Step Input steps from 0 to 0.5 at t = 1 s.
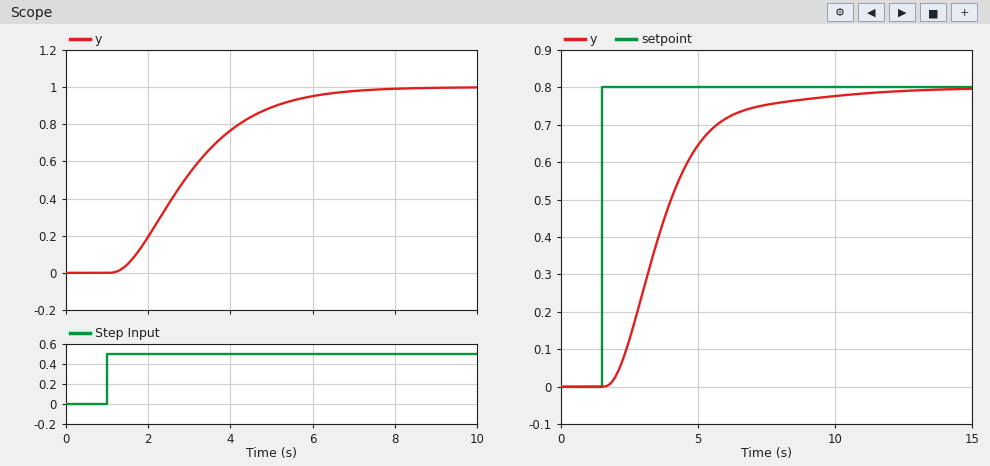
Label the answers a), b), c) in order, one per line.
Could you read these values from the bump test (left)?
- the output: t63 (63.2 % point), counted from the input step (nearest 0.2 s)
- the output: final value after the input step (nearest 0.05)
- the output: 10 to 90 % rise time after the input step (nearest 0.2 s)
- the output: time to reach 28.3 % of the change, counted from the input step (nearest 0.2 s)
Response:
a) 2.4 s
b) 1.00
c) 3.4 s
d) 1.2 s
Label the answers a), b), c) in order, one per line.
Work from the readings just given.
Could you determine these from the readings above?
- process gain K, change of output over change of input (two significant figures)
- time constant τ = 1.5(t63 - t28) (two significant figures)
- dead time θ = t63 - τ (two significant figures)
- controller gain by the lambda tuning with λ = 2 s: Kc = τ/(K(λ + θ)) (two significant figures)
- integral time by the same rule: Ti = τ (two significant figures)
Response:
a) 2.0
b) 1.8 s
c) 0.60 s
d) 0.35
e) 1.8 s
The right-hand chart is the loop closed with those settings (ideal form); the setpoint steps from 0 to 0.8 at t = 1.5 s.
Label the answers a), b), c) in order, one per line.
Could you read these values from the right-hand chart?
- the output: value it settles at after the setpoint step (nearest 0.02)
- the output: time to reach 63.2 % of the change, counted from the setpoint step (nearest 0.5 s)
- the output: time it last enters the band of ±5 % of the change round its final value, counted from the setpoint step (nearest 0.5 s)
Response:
a) 0.80
b) 2.5 s
c) 6.5 s
